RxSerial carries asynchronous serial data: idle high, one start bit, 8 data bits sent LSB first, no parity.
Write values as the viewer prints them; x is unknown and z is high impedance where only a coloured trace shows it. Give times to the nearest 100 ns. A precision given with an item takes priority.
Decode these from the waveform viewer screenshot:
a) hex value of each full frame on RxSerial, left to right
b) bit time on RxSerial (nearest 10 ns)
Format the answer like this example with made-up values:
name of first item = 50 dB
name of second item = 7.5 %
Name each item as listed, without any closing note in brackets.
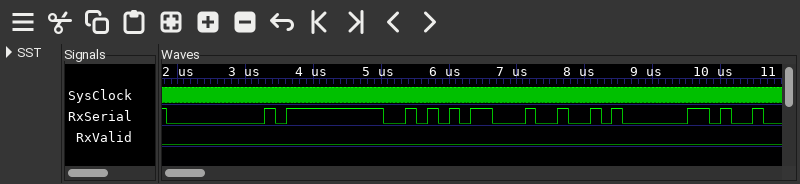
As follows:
hex value of each full frame on RxSerial, left to right = 00, FF, AA, 24, 81
bit time on RxSerial = 160 ns
